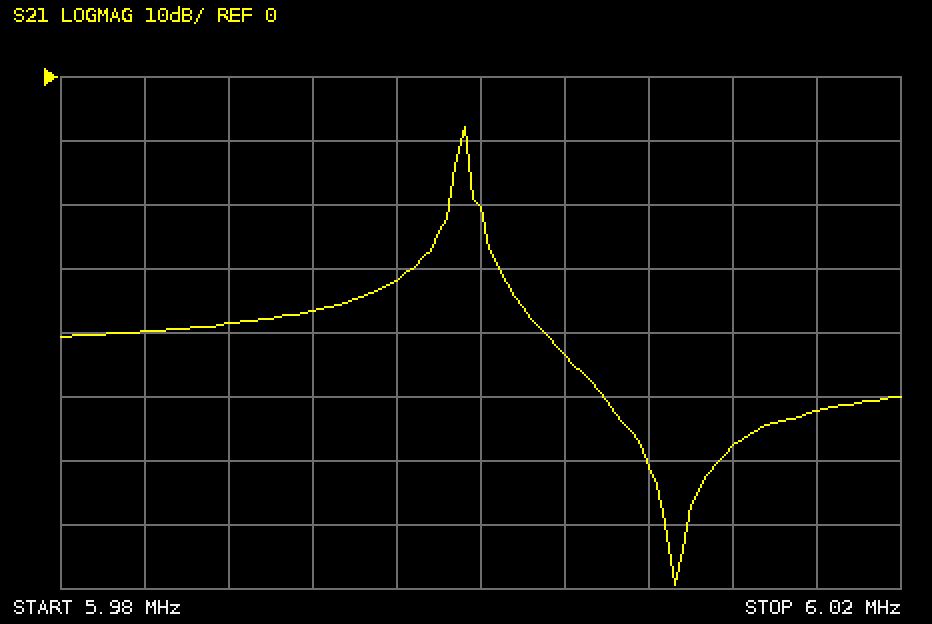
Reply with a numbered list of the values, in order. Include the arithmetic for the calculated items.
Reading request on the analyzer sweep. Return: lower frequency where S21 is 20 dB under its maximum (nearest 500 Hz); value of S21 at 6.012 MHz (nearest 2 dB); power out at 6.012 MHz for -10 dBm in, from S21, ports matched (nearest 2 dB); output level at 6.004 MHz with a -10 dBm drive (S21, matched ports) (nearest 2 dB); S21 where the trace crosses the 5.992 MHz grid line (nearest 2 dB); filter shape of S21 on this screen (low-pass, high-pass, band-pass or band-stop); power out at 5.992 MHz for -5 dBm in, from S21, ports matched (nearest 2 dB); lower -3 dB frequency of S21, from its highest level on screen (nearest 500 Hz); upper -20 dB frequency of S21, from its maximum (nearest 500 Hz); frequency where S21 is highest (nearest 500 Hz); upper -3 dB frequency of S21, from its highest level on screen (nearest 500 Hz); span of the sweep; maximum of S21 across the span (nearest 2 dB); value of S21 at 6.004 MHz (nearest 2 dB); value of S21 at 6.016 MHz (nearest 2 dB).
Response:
1. 5.9975 MHz
2. -58 dB
3. -10 dBm + (-58 dB) = -68 dBm
4. -10 dBm + (-44 dB) = -54 dBm
5. -36 dB
6. band-pass
7. -5 dBm + (-36 dB) = -42 dBm
8. 5.9990 MHz
9. 6.0005 MHz
10. 5.9990 MHz
11. 5.9995 MHz
12. 40 kHz
13. -8 dB
14. -44 dB
15. -52 dB
